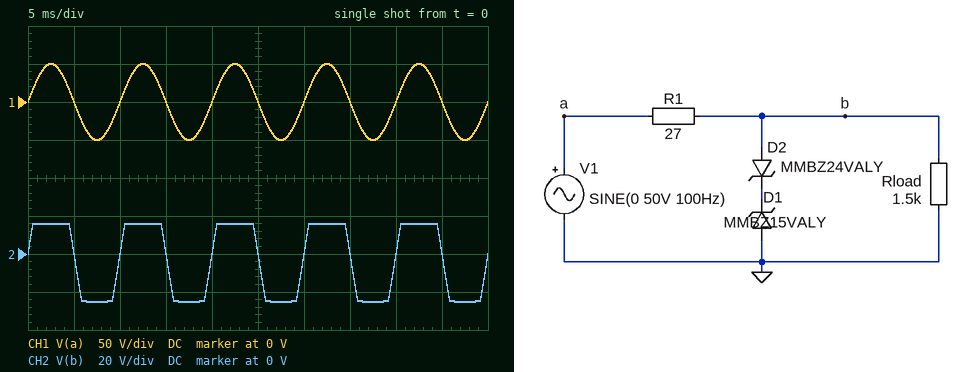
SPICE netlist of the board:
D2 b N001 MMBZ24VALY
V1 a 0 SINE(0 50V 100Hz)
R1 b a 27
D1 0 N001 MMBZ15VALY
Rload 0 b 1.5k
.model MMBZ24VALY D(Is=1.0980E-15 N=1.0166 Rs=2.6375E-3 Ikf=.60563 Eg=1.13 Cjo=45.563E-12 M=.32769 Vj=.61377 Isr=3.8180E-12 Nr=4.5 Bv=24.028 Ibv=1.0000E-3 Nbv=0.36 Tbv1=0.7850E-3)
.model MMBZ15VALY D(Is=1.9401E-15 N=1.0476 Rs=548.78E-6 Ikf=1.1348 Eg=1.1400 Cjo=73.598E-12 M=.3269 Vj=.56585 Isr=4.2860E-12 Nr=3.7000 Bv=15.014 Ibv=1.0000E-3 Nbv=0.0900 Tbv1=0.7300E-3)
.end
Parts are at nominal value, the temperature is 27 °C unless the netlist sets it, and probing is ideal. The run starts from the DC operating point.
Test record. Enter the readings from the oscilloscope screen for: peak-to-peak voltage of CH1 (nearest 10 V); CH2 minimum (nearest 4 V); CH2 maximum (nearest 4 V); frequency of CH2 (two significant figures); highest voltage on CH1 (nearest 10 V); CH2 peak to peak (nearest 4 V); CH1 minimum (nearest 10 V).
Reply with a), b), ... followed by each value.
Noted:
a) 100 V
b) -24 V
c) 16 V
d) 100 Hz
e) 50 V
f) 40 V
g) -50 V
